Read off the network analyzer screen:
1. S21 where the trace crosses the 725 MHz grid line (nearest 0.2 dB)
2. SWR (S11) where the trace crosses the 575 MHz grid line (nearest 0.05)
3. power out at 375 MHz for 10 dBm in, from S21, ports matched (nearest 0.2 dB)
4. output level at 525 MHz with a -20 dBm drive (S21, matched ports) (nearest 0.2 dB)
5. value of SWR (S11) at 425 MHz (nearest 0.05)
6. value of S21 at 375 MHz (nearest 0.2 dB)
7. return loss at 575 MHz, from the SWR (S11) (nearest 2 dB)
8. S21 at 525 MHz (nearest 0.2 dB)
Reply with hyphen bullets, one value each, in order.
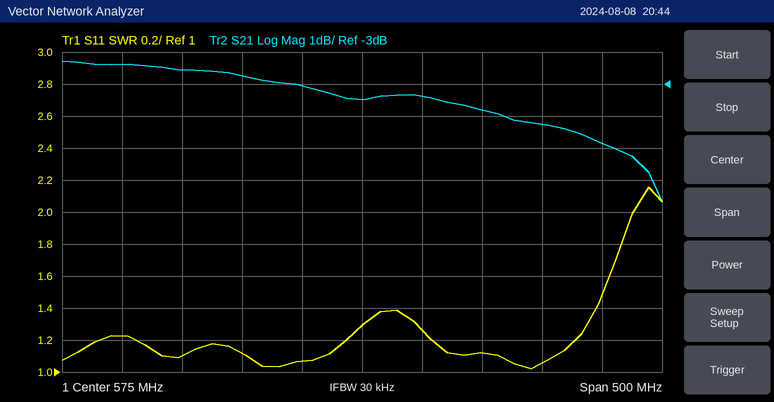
- -4.2 dB
- 1.30
- 7.6 dBm
- -23.0 dBm
- 1.10
- -2.4 dB
- 18 dB
- -3.0 dB
